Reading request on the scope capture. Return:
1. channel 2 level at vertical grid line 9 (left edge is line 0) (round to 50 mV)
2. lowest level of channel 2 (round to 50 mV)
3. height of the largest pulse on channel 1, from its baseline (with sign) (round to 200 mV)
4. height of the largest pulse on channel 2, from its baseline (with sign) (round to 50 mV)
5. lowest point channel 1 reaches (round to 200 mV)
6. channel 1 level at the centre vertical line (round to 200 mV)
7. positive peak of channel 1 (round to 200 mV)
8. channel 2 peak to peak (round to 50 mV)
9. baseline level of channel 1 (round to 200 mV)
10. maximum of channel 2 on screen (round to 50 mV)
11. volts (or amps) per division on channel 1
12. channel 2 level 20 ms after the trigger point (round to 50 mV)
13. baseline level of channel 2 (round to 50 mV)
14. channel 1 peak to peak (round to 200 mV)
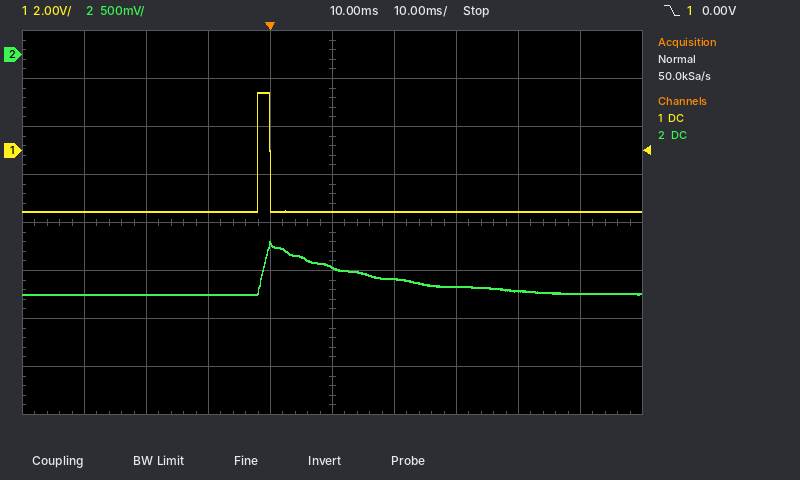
-2.50 V
-2.50 V
+5.0 V
+550 mV
-2.6 V
-2.6 V
2.4 V
550 mV
-2.6 V
-1.95 V
2 V
-2.35 V
-2.50 V
5.0 V
